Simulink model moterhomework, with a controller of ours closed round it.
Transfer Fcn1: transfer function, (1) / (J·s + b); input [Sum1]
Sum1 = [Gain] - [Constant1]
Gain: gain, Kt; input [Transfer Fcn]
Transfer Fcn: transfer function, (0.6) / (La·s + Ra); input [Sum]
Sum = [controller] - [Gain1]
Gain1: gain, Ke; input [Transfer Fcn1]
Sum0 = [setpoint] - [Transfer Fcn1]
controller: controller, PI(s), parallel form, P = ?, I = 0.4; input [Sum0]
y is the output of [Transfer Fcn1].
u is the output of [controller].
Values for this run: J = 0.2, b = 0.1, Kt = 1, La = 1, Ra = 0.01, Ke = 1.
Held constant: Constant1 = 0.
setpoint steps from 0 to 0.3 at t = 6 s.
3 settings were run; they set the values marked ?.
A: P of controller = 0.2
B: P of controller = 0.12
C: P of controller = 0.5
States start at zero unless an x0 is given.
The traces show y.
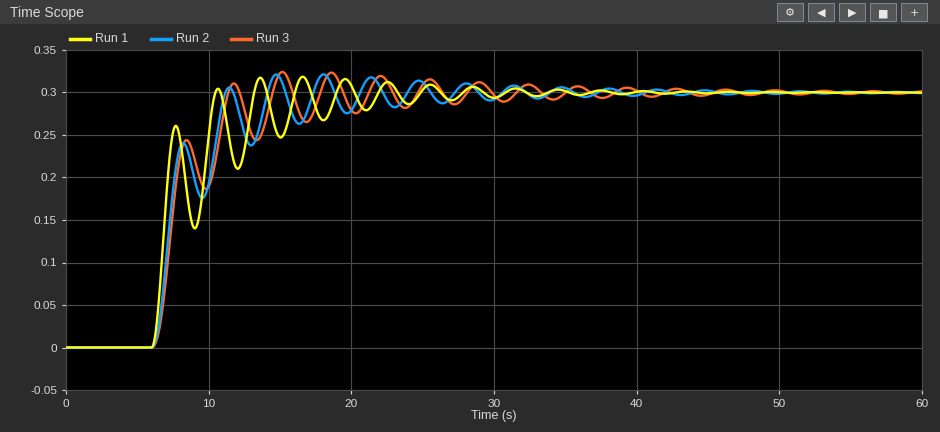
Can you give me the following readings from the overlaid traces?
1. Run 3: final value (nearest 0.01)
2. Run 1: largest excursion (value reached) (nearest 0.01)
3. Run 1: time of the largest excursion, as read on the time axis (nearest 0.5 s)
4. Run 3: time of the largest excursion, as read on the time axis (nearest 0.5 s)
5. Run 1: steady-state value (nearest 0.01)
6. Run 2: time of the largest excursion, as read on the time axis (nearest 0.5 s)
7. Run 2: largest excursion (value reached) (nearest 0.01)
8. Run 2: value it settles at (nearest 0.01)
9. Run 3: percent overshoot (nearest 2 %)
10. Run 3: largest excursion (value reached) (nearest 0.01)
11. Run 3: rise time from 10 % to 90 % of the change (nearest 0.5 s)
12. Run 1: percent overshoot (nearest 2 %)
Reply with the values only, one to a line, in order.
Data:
0.30
0.32
16.5 s
15.0 s
0.30
18.0 s
0.32
0.30
8 %
0.32
4.5 s
6 %
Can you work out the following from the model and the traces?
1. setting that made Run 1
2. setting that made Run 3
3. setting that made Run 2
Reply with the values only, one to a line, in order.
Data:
C
B
A
